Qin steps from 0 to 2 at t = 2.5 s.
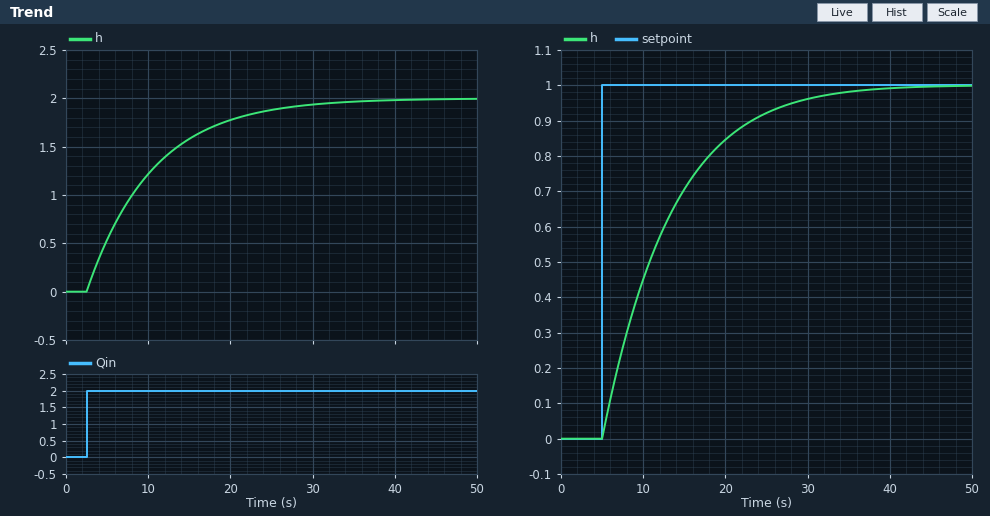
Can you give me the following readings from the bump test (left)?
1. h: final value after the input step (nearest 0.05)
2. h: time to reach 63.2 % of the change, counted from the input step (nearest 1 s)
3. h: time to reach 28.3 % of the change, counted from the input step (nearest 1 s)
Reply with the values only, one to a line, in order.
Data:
2.00
8 s
3 s
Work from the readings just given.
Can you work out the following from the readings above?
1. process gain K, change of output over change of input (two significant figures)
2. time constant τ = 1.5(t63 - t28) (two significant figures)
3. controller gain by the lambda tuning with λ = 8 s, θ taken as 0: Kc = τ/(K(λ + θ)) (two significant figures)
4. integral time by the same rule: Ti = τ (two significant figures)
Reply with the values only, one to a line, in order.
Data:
1.0
7.5 s
0.94
7.5 s
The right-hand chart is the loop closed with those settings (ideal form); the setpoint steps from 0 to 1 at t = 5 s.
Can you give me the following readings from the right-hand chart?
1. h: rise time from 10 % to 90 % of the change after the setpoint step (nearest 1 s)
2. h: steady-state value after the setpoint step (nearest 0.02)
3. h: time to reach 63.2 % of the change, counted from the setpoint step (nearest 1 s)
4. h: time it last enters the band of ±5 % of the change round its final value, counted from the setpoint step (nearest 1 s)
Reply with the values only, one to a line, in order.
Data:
17 s
1.00
8 s
23 s
